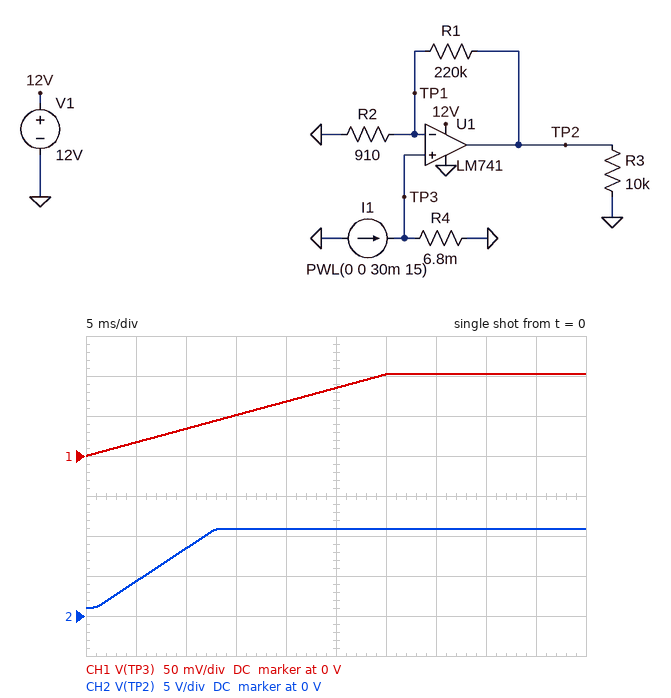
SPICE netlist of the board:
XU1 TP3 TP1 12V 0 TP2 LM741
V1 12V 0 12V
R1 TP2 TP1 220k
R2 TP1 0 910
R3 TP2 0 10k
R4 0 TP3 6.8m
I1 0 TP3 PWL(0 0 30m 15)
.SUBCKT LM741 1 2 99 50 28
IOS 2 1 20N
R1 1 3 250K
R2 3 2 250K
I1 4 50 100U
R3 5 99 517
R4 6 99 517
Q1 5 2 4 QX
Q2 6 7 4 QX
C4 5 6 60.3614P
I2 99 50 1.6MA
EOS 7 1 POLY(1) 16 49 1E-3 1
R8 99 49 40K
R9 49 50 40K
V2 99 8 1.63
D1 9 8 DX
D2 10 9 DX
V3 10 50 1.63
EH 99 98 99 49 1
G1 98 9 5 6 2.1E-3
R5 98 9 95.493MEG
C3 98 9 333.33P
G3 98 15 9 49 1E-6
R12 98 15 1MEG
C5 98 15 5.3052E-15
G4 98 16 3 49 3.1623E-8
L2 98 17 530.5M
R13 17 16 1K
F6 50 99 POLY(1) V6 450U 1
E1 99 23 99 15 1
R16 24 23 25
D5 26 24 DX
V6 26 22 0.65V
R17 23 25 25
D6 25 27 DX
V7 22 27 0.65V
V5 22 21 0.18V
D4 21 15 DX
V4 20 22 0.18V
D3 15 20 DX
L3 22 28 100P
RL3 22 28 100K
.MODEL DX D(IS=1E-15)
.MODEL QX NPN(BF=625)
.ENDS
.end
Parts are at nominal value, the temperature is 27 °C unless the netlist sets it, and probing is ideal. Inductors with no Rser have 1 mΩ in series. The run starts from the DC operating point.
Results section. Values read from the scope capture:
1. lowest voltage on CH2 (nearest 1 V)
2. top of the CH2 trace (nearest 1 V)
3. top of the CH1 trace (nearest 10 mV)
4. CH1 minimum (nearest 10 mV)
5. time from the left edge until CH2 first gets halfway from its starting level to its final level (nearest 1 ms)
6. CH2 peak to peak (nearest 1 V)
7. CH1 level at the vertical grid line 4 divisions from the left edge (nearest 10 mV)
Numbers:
1 V
11 V
100 mV
0 V
7 ms
10 V
70 mV
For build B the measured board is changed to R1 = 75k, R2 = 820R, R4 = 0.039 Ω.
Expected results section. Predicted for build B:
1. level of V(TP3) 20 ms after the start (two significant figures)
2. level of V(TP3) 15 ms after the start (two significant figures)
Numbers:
390 mV
290 mV
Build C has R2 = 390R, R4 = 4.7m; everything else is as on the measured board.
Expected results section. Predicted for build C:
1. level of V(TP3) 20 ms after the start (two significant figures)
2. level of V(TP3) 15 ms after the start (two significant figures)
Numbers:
47 mV
35 mV
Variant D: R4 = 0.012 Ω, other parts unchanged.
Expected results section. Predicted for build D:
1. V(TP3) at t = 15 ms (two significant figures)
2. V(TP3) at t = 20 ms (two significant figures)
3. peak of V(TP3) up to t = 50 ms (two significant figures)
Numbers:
90 mV
120 mV
180 mV
